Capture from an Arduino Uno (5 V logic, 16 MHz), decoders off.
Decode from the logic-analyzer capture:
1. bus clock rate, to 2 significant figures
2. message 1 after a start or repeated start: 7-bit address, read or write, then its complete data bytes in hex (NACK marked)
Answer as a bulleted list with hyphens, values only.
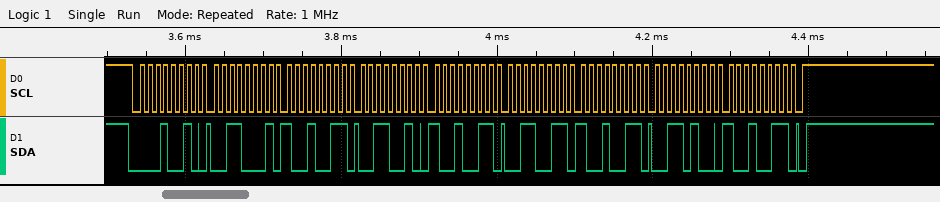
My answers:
- 100 kHz
- 0x09 write: 31 93 32 93 33 93 34 93
